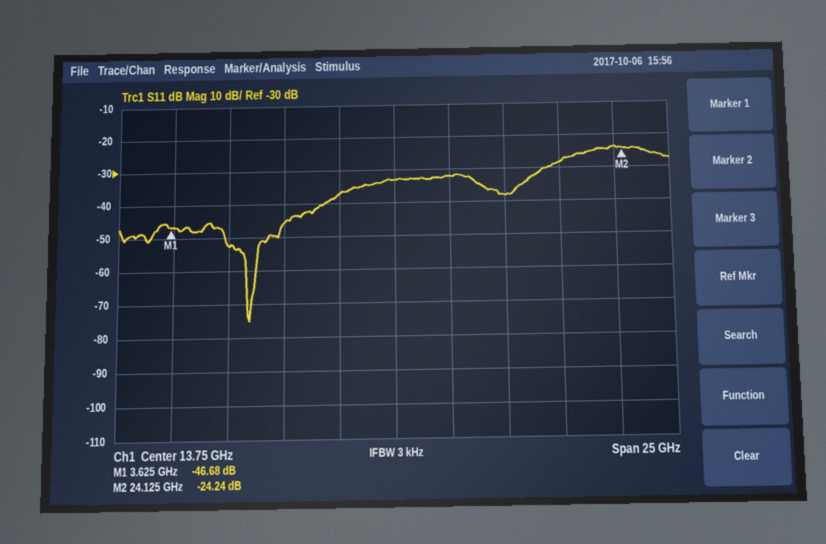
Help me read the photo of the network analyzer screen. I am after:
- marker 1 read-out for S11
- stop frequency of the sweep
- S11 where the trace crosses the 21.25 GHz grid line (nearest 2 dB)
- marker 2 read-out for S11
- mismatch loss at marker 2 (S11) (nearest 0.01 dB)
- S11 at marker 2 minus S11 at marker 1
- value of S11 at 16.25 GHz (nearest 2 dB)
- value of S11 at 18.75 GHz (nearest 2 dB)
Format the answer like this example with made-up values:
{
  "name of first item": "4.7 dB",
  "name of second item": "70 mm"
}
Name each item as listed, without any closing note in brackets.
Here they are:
{
  "marker 1 read-out for S11": "-46.68 dB",
  "stop frequency of the sweep": "26.25 GHz",
  "S11 where the trace crosses the 21.25 GHz grid line": "-28 dB",
  "marker 2 read-out for S11": "-24.24 dB",
  "mismatch loss at marker 2 (S11)": "0.02 dB",
  "S11 at marker 2 minus S11 at marker 1": "22.44 dB",
  "value of S11 at 16.25 GHz": "-32 dB",
  "value of S11 at 18.75 GHz": "-38 dB"
}
